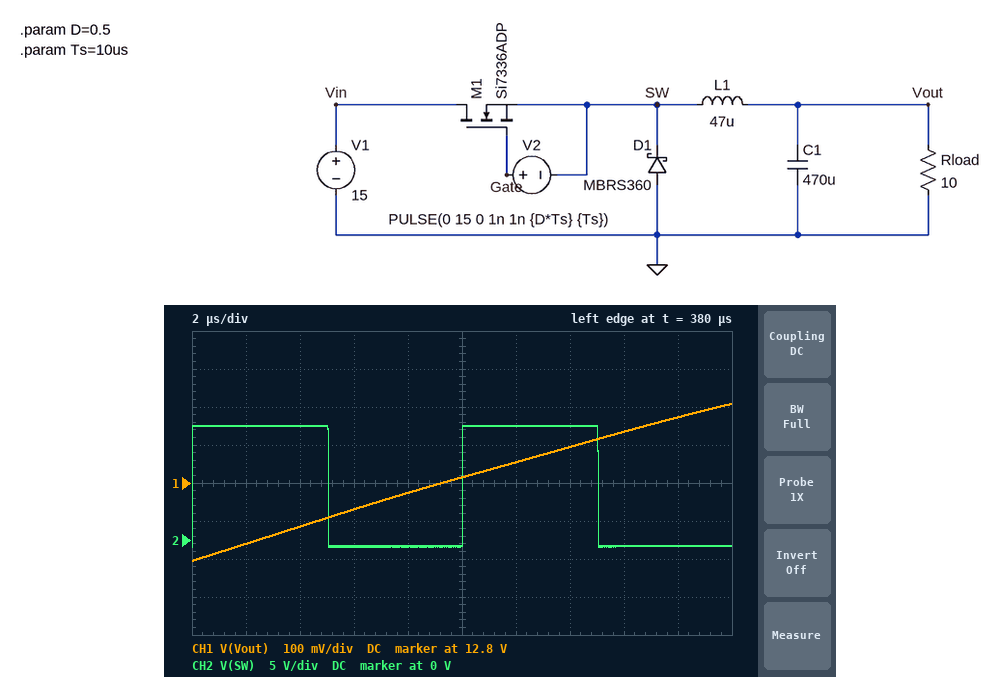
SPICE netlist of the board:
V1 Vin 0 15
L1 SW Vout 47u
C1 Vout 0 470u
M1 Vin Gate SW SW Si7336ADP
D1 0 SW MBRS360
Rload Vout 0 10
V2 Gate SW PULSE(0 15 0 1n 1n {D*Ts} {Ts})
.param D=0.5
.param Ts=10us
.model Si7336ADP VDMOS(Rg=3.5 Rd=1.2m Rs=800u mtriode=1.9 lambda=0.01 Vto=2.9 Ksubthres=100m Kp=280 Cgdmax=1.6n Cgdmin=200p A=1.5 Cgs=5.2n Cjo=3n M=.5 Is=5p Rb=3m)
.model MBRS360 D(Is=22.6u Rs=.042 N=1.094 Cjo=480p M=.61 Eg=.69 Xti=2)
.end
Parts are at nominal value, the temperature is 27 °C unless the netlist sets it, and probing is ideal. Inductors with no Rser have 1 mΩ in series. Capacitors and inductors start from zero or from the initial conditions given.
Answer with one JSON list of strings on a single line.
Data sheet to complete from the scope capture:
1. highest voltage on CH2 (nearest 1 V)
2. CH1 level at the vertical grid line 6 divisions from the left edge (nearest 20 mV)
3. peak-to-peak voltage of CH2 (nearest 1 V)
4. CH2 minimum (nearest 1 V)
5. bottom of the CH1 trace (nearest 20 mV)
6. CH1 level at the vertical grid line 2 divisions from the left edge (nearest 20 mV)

["15 V", "12.86 V", "16 V", "-1 V", "12.60 V", "12.68 V"]
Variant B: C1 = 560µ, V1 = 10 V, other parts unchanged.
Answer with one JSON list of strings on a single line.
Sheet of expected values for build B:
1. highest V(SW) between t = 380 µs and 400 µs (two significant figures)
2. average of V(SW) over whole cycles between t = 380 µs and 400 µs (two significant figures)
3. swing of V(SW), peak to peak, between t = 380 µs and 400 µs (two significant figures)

["10 V", "4.6 V", "11 V"]
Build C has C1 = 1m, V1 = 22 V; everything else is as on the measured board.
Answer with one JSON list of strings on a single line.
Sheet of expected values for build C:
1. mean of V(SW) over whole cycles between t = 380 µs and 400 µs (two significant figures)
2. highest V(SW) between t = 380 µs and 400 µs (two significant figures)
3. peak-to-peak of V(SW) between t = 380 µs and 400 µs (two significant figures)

["9.9 V", "22 V", "24 V"]
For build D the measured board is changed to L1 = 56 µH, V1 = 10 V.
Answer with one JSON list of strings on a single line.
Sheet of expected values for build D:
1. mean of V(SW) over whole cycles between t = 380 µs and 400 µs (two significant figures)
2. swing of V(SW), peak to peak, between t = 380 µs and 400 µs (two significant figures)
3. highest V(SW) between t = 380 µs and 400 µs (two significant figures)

["4.7 V", "11 V", "10 V"]
